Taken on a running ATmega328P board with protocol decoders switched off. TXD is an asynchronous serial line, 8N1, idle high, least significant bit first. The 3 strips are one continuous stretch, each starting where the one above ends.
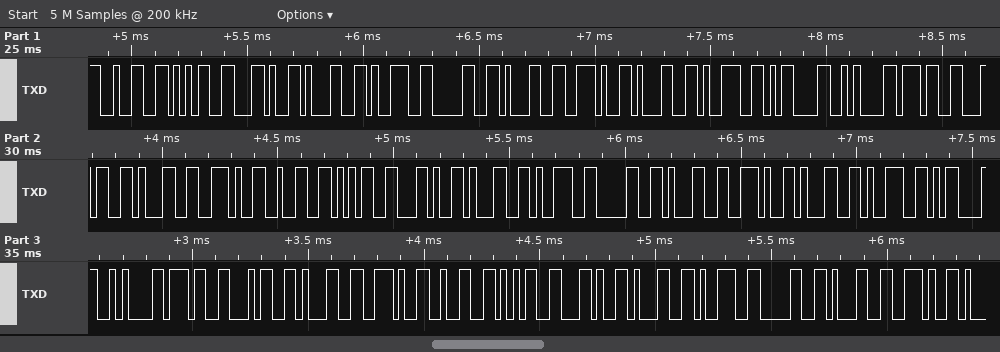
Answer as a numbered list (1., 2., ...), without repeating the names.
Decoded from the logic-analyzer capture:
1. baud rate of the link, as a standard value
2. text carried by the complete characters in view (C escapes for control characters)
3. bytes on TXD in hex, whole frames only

1. 38400 baud
2. "25,1901.19\r\n741.25,1901.19\r\n741.25,1901."
3. 32 35 2C 31 39 30 31 2E 31 39 0D 0A 37 34 31 2E 32 35 2C 31 39 30 31 2E 31 39 0D 0A 37 34 31 2E 32 35 2C 31 39 30 31 2E
